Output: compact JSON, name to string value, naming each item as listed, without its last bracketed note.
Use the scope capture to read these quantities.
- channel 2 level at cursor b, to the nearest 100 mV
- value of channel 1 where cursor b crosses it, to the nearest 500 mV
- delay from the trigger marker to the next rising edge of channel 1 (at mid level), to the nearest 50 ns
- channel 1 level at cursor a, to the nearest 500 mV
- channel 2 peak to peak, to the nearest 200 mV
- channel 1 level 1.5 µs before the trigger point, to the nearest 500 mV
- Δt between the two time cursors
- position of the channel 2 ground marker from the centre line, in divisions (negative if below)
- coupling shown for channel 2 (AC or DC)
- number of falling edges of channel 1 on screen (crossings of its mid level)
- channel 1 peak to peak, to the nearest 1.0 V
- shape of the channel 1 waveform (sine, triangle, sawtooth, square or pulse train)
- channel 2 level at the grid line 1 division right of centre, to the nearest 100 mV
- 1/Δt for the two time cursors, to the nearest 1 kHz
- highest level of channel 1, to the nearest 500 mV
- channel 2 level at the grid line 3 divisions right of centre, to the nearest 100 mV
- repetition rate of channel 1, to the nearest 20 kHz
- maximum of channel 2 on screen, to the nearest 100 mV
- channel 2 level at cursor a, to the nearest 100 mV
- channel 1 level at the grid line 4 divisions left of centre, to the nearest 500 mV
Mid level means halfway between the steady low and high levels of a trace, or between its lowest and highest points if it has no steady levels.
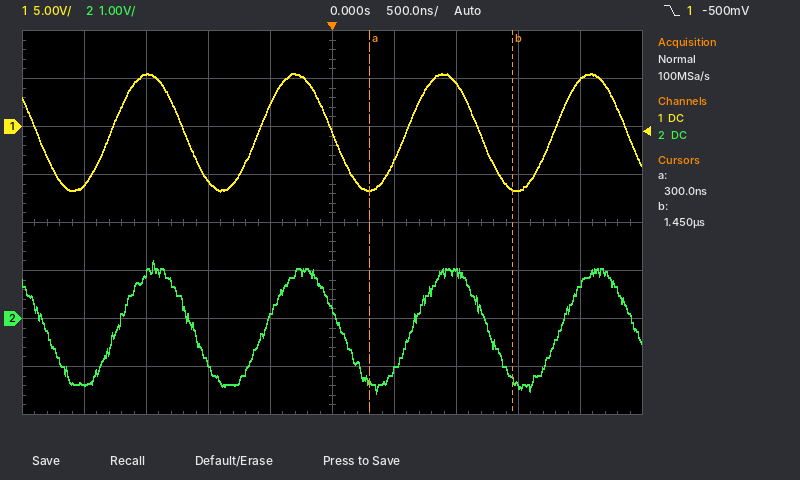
{"channel 2 level at cursor b, to the nearest 100 mV": "-1.3 V", "value of channel 1 where cursor b crosses it, to the nearest 500 mV": "-6.5 V", "delay from the trigger marker to the next rising edge of channel 1 (at mid level), to the nearest 50 ns": "600 ns", "channel 1 level at cursor a, to the nearest 500 mV": "-6.5 V", "channel 2 peak to peak, to the nearest 200 mV": "2.8 V", "channel 1 level 1.5 µs before the trigger point, to the nearest 500 mV": "5.5 V", "Δt between the two time cursors": "1.15 µs", "position of the channel 2 ground marker from the centre line, in divisions": "-2.0 div", "coupling shown for channel 2": "DC", "number of falling edges of channel 1 on screen": "5", "channel 1 peak to peak, to the nearest 1.0 V": "12.0 V", "shape of the channel 1 waveform": "sine", "channel 2 level at the grid line 1 division right of centre, to the nearest 100 mV": "-1.1 V", "1/Δt for the two time cursors, to the nearest 1 kHz": "870 kHz", "highest level of channel 1, to the nearest 500 mV": "5.5 V", "channel 2 level at the grid line 3 divisions right of centre, to the nearest 100 mV": "-1.4 V", "repetition rate of channel 1, to the nearest 20 kHz": "840 kHz", "maximum of channel 2 on screen, to the nearest 100 mV": "1.2 V", "channel 2 level at cursor a, to the nearest 100 mV": "-1.3 V", "channel 1 level at the grid line 4 divisions left of centre, to the nearest 500 mV": "-6.0 V"}
